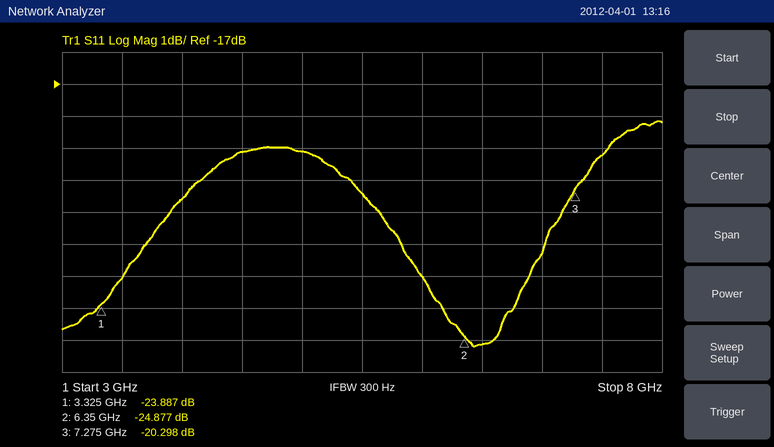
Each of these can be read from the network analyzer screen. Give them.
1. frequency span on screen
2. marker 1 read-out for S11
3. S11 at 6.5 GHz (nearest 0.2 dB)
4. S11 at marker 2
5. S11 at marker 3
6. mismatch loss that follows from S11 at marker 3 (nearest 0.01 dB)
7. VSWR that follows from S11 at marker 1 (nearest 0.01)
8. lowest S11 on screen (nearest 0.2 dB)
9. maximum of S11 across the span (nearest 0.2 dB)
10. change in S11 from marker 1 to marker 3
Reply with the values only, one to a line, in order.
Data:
5 GHz
-23.887 dB
-25.2 dB
-24.877 dB
-20.298 dB
0.04 dB
1.14
-25.2 dB
-18.2 dB
3.589 dB
